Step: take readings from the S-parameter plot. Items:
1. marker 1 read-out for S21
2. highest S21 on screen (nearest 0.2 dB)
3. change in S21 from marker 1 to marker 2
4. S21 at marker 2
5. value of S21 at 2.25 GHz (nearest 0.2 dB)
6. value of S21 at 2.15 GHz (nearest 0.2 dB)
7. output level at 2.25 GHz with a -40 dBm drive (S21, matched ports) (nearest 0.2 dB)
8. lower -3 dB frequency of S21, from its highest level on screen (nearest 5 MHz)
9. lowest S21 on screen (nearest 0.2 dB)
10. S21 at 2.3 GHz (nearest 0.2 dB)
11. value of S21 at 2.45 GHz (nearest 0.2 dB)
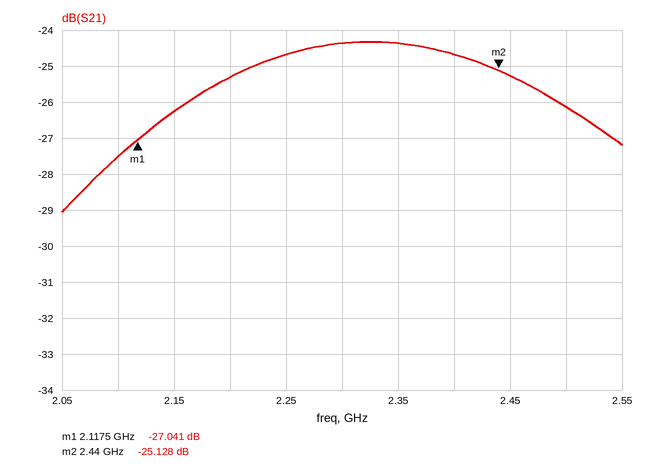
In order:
-27.041 dB
-24.4 dB
1.913 dB
-25.128 dB
-24.6 dB
-26.2 dB
-64.6 dBm
2.105 GHz
-29.0 dB
-24.4 dB
-25.2 dB
